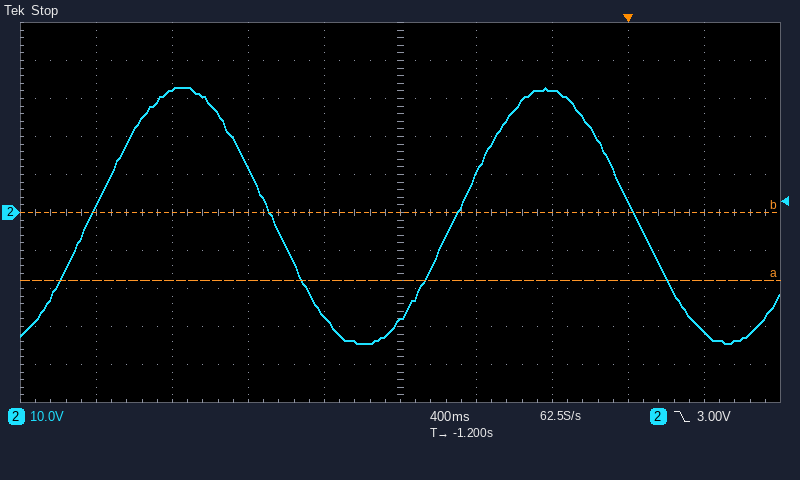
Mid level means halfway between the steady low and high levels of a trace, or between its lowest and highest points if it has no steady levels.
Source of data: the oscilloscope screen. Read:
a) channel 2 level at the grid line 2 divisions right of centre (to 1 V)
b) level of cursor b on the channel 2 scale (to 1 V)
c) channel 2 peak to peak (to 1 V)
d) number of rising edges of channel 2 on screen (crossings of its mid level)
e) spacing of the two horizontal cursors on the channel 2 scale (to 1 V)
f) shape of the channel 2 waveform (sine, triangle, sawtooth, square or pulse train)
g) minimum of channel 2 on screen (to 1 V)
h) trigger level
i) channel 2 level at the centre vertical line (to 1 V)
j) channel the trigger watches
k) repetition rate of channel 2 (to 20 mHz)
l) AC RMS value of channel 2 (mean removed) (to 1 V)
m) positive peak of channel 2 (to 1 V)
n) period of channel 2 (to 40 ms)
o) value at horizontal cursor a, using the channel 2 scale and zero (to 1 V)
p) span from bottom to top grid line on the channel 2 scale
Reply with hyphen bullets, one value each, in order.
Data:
- 32 V
- 0 V
- 67 V
- 2
- 18 V
- sine
- -34 V
- 3.00 V
- -28 V
- channel 2
- 520 mHz
- 24 V
- 33 V
- 1.92 s
- -18 V
- 100 V
